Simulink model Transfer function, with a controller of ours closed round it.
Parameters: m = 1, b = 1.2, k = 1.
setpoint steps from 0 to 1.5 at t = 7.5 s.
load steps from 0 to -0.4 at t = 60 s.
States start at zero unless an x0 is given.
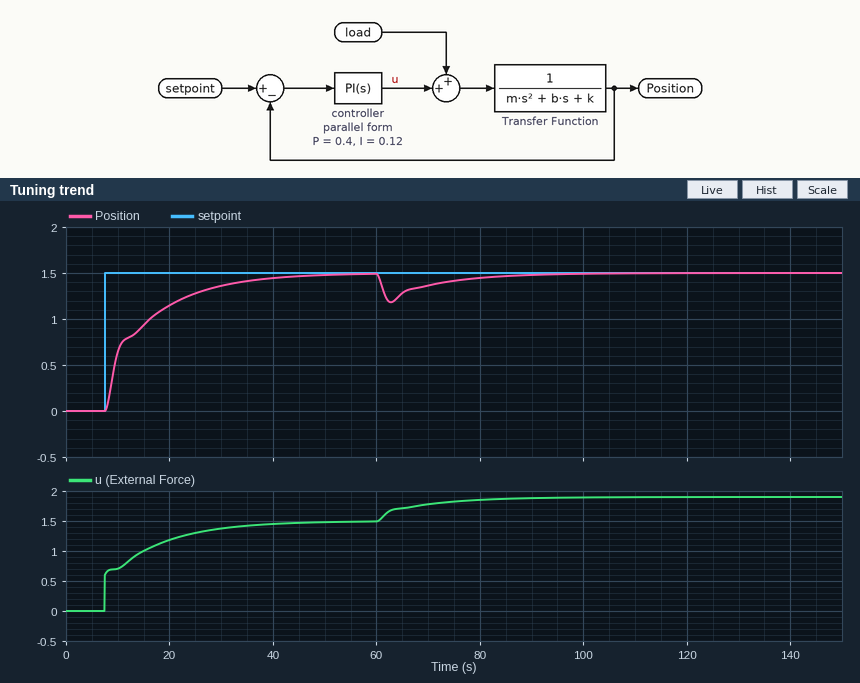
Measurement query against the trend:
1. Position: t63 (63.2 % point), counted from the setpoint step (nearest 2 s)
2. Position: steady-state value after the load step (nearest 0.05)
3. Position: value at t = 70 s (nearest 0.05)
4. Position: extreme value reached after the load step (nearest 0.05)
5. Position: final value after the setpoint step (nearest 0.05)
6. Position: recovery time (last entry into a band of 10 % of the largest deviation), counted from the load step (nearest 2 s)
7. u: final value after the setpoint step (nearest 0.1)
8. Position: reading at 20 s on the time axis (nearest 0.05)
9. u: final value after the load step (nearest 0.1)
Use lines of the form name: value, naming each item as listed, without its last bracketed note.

Position: t63 (63.2 % point), counted from the setpoint step: 8 s
Position: steady-state value after the load step: 1.50
Position: value at t = 70 s: 1.35
Position: extreme value reached after the load step: 1.20
Position: final value after the setpoint step: 1.50
Position: recovery time (last entry into a band of 10 % of the largest deviation), counted from the load step: 26 s
u: final value after the setpoint step: 1.5
Position: reading at 20 s on the time axis: 1.15
u: final value after the load step: 1.9
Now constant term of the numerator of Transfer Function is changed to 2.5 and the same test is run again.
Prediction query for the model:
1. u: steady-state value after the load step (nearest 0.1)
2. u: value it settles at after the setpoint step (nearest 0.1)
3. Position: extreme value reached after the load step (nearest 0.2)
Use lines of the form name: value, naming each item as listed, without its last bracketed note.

u: steady-state value after the load step: 1.0
u: value it settles at after the setpoint step: 0.6
Position: extreme value reached after the load step: 1.0
